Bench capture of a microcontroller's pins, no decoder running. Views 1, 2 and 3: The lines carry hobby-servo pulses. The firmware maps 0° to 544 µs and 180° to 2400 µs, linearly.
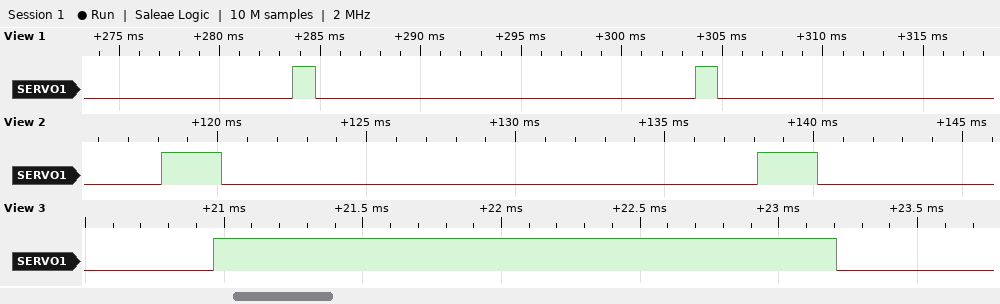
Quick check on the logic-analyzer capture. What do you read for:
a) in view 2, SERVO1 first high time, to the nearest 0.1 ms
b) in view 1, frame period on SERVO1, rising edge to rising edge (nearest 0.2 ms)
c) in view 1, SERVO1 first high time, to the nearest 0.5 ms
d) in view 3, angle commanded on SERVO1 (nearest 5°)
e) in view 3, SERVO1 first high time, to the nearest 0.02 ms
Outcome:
2.0 ms
20.0 ms
1.0 ms
165°
2.24 ms
